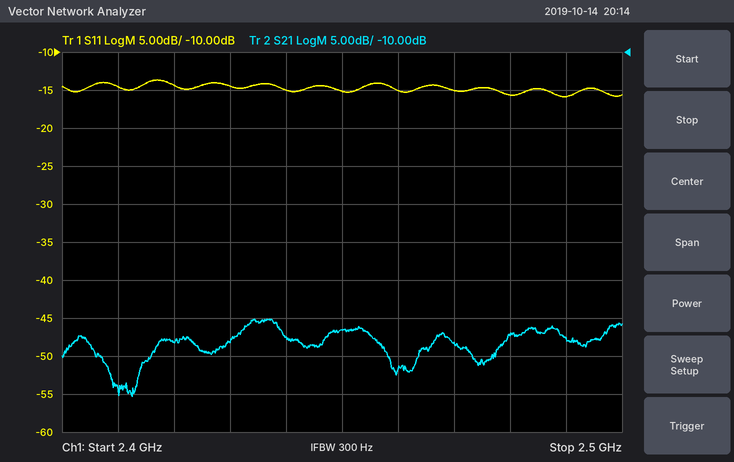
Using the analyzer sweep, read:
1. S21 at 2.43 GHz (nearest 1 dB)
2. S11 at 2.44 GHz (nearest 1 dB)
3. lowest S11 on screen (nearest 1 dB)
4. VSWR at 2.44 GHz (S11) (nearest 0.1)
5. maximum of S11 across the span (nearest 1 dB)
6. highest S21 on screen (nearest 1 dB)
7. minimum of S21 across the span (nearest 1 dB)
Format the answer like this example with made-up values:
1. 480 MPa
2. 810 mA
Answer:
1. -48 dB
2. -15 dB
3. -16 dB
4. 1.4
5. -14 dB
6. -45 dB
7. -55 dB
